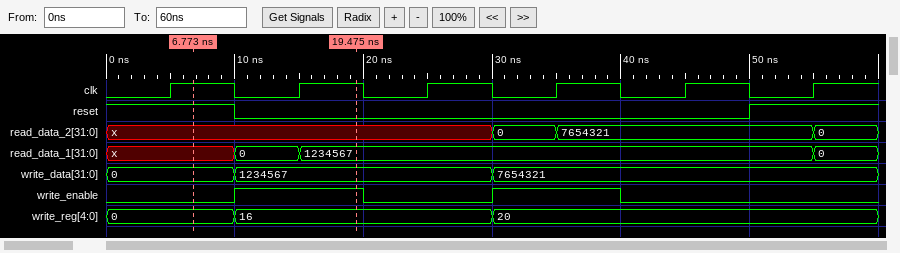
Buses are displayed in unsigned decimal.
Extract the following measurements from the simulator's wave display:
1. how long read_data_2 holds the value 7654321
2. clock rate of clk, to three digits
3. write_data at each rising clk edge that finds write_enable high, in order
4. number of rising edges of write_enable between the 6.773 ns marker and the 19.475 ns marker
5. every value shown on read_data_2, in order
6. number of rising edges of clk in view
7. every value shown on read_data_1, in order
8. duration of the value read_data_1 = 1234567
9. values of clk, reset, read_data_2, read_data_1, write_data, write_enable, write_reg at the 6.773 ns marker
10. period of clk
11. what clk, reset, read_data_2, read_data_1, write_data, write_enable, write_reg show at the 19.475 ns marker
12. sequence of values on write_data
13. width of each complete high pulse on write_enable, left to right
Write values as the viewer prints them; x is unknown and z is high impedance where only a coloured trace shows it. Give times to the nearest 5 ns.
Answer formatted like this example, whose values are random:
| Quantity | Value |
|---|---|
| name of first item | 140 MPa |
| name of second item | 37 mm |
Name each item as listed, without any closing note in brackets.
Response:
| Quantity | Value |
|---|---|
| how long read_data_2 holds the value 7654321 | 20 ns |
| clock rate of clk, to three digits | 100 MHz |
| write_data at each rising clk edge that finds write_enable high, in order | 1234567, 7654321 |
| number of rising edges of write_enable between the 6.773 ns marker and the 19.475 ns marker | 1 |
| every value shown on read_data_2, in order | x, 0, 7654321, 0 |
| number of rising edges of clk in view | 6 |
| every value shown on read_data_1, in order | x, 0, 1234567, 0 |
| duration of the value read_data_1 = 1234567 | 40 ns |
| values of clk, reset, read_data_2, read_data_1, write_data, write_enable, write_reg at the 6.773 ns marker | clk=1, reset=1, read_data_2=x, read_data_1=x, write_data=0, write_enable=0, write_reg=0 |
| period of clk | 10 ns |
| what clk, reset, read_data_2, read_data_1, write_data, write_enable, write_reg show at the 19.475 ns marker | clk=1, reset=0, read_data_2=x, read_data_1=1234567, write_data=1234567, write_enable=1, write_reg=16 |
| sequence of values on write_data | 0, 1234567, 7654321 |
| width of each complete high pulse on write_enable, left to right | 10 ns, 10 ns |
